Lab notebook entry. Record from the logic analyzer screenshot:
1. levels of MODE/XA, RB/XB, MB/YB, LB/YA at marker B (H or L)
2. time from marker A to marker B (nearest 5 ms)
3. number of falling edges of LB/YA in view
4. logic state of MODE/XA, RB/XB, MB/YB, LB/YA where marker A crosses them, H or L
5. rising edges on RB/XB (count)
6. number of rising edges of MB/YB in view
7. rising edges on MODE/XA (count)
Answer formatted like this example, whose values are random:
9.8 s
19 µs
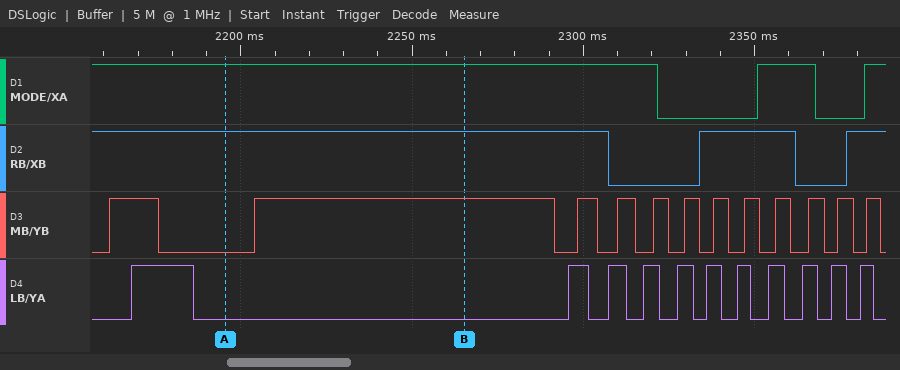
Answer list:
MODE/XA=H, RB/XB=H, MB/YB=H, LB/YA=L
70 ms
11
MODE/XA=H, RB/XB=H, MB/YB=L, LB/YA=L
2
12
2
